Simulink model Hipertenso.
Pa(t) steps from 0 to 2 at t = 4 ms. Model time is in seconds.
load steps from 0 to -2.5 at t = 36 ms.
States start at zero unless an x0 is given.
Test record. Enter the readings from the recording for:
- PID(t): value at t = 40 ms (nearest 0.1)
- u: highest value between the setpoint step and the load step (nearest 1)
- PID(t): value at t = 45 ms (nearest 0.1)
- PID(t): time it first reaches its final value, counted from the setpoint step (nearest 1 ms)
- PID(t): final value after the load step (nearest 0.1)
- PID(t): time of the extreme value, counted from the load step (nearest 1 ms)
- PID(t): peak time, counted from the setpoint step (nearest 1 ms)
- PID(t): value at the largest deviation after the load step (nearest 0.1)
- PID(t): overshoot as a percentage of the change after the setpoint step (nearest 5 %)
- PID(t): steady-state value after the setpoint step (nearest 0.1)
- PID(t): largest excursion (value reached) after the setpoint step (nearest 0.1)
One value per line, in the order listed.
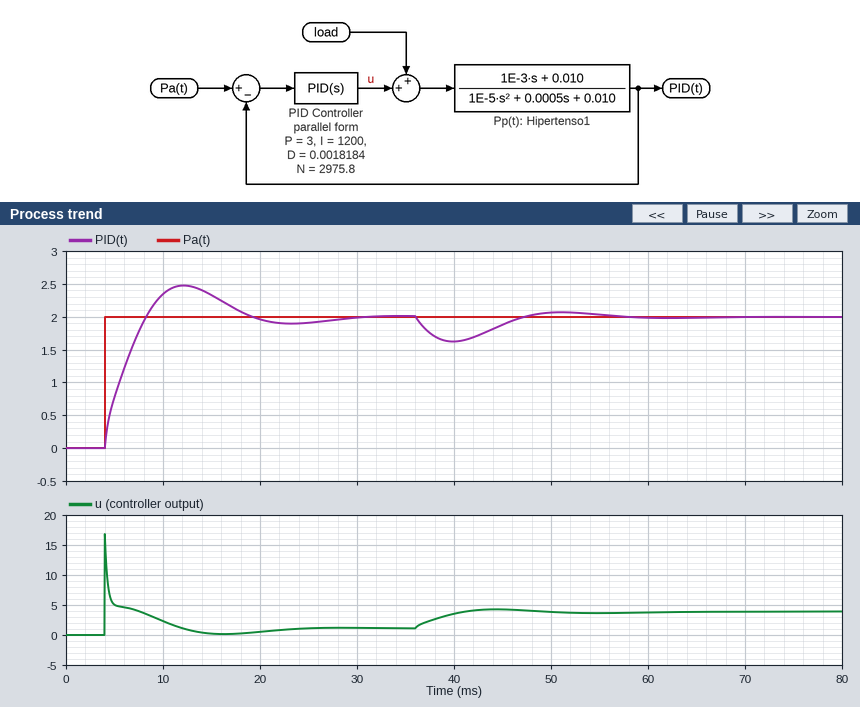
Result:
1.6
17
1.9
4 ms
2.0
4 ms
8 ms
1.6
25 %
2.0
2.5
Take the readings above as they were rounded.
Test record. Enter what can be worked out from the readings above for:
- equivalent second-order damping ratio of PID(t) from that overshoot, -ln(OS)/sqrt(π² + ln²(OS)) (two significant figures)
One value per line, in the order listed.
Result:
0.40
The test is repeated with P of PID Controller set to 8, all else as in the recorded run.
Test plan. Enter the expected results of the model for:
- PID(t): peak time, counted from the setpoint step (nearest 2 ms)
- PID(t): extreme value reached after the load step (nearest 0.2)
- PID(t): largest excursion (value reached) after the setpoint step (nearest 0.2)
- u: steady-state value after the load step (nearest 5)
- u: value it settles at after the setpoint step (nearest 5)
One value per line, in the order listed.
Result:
6 ms
1.8
2.2
5
0
